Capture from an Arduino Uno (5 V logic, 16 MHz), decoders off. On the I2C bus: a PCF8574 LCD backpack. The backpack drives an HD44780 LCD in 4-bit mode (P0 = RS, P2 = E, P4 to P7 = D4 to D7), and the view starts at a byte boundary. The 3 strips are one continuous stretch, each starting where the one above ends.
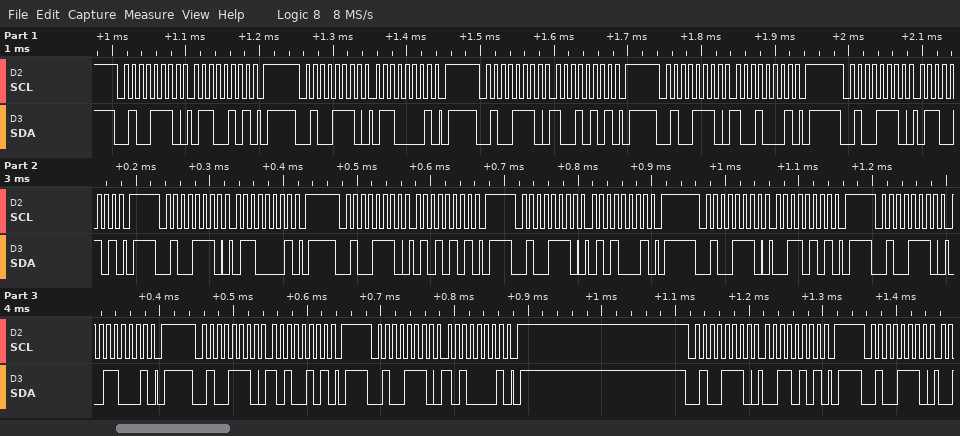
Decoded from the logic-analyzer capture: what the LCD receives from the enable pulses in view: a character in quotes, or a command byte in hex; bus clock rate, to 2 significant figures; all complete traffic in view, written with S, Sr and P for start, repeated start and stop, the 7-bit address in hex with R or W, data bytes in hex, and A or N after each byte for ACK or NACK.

'i' 'e' ':'
100 kHz
S 27W A 65 A P S 27W A 61 A P S 27W A 95 A P S 27W A 91 A P S 27W A 65 A P S 27W A 61 A P S 27W A 55 A P S 27W A 51 A P S 27W A 35 A P S 27W A 31 A P S 27W A A5 A P S 27W A A1 A P S 27W A 35 A P S 27W A
